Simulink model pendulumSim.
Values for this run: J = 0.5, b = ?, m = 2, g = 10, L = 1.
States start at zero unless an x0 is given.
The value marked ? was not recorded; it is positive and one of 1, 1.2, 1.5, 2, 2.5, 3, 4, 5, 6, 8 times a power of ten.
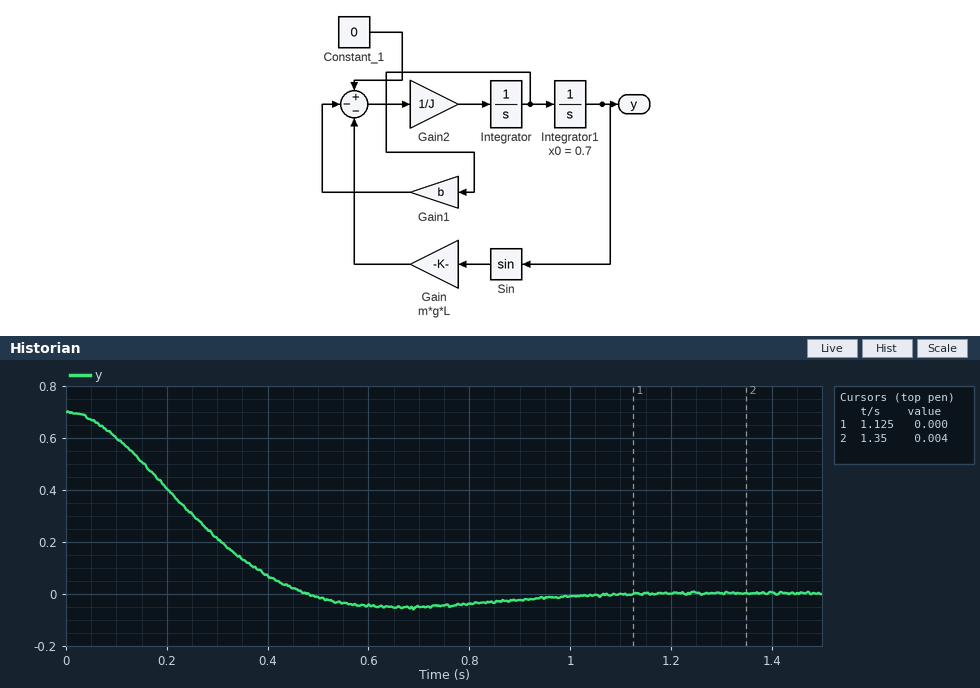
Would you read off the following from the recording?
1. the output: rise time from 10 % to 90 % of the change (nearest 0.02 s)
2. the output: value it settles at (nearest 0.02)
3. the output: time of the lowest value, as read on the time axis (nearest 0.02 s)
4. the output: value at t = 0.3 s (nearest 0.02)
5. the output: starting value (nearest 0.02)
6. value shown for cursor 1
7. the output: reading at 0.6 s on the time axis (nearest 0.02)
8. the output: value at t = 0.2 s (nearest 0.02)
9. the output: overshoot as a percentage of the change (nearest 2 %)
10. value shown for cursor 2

0.32 s
0.00
0.66 s
0.22
0.70
0.000
-0.04
0.40
8 %
0.004
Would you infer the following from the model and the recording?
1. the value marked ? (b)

4
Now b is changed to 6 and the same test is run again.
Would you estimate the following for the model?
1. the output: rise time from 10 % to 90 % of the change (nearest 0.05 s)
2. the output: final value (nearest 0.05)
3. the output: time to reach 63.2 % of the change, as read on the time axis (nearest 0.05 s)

0.50 s
0.00
0.35 s
